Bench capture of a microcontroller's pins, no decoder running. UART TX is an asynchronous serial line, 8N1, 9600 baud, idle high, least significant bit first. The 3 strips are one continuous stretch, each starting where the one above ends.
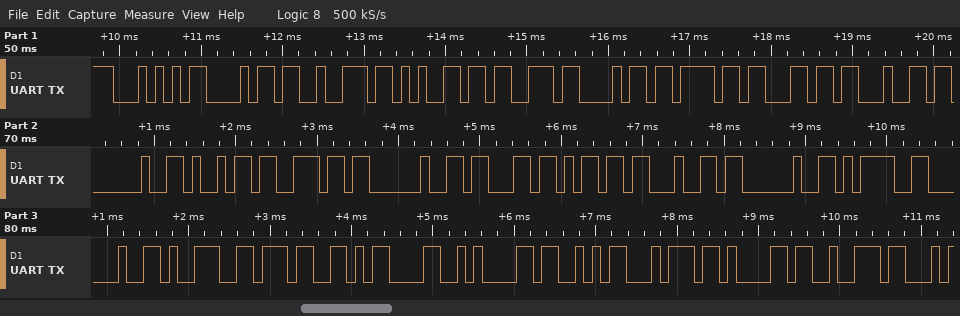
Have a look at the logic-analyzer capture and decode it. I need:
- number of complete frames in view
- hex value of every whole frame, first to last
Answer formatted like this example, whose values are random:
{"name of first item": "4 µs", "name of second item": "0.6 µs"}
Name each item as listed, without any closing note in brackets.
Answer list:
{"number of complete frames in view": "27", "hex value of every whole frame, first to last": "54 68 72 65 73 68 6F 6C 64 20 69 6E 20 63 6D 64 20 3D 20 39 37 0D 0A 53 74 61 72"}
